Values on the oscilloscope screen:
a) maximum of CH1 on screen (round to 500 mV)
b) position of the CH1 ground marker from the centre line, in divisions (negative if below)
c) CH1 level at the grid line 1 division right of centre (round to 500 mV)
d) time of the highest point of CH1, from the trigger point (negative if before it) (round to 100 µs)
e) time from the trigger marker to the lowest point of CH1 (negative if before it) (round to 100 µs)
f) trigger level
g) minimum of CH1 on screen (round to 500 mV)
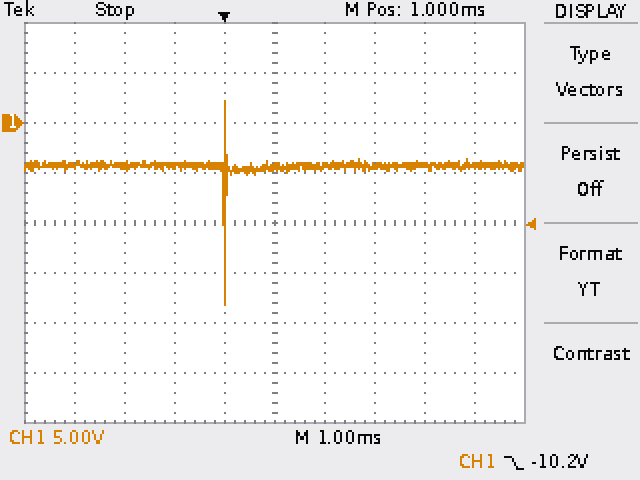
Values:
2.0 V
+2.0 div
-4.5 V
0.0 ms
0.0 ms
-10.2 V
-18.0 V
